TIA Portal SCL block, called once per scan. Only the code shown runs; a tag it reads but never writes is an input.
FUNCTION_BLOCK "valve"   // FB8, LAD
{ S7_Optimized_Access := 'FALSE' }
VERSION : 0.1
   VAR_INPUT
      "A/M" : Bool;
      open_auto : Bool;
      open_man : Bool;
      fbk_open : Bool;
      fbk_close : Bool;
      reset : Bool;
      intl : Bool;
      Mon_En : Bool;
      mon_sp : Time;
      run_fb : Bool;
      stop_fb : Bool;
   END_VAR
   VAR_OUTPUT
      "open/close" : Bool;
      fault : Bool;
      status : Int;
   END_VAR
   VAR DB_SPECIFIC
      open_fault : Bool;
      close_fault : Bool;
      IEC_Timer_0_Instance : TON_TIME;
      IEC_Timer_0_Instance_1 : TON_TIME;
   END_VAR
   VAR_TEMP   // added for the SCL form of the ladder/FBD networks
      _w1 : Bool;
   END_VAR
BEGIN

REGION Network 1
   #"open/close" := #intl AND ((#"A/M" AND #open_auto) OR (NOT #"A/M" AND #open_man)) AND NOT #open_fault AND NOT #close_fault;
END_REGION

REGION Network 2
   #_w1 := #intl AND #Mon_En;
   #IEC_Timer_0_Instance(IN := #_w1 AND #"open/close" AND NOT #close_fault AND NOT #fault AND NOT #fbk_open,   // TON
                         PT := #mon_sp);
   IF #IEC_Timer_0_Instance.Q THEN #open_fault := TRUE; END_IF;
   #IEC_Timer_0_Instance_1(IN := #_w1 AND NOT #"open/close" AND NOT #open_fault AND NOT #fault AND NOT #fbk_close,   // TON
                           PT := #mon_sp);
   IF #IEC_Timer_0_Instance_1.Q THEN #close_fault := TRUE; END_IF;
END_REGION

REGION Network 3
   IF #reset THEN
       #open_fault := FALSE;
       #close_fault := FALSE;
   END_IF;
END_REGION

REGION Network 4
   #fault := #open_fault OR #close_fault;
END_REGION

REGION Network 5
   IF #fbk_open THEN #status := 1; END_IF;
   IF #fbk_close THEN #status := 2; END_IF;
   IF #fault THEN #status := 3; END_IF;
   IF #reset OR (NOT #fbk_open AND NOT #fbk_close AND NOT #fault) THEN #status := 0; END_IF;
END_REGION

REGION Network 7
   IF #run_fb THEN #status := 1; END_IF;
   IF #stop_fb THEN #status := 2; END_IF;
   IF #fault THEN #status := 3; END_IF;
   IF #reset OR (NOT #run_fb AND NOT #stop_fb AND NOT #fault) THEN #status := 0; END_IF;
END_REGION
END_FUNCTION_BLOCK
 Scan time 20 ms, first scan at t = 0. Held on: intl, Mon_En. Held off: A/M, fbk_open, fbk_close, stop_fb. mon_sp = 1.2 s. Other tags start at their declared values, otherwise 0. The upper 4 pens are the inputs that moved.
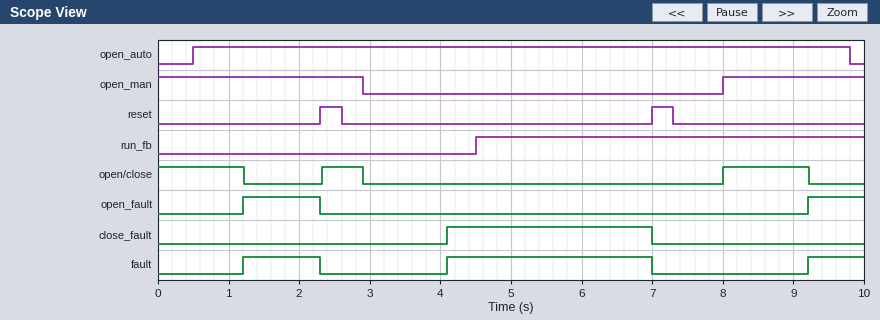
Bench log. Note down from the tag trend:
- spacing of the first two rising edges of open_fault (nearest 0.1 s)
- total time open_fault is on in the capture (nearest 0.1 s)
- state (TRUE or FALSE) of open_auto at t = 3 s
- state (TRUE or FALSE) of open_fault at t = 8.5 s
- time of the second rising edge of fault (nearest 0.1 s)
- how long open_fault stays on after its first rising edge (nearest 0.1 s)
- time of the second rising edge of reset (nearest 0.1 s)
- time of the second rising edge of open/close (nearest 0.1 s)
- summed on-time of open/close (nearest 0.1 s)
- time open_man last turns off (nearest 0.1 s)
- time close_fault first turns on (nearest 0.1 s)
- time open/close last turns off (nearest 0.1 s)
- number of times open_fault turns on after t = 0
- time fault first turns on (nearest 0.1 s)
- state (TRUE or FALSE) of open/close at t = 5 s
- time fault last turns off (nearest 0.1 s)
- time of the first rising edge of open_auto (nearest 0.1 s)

8.0 s
1.9 s
TRUE
FALSE
4.1 s
1.1 s
7.0 s
8.0 s
3.0 s
2.9 s
4.1 s
9.2 s
2
1.2 s
FALSE
7.0 s
0.5 s
